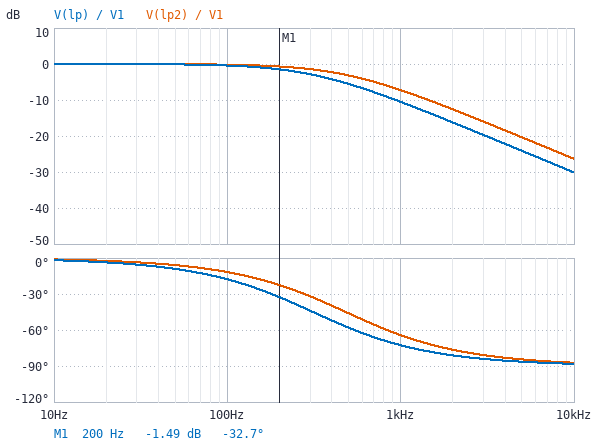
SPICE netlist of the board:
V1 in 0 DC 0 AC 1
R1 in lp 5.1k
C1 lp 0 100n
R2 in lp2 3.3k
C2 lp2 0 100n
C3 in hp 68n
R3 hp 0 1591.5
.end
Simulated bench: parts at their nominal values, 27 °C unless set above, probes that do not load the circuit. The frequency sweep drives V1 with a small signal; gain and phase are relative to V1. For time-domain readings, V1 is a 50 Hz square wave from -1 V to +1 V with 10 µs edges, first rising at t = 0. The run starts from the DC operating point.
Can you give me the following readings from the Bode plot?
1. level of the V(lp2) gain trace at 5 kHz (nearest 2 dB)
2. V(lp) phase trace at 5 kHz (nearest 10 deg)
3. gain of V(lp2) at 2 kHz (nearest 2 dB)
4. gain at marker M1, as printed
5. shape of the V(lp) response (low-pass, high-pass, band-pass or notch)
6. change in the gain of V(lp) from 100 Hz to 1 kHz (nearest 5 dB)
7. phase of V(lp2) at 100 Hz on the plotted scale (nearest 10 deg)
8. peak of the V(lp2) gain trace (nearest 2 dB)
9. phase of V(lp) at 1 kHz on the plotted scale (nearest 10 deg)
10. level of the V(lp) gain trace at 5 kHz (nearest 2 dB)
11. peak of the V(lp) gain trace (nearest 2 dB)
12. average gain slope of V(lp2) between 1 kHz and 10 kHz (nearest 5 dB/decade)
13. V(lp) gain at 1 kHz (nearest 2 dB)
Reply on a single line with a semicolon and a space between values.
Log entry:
-20 dB; -90 deg; -12 dB; -1.49 dB; low-pass; -10 dB; -10 deg; 0 dB; -70 deg; -24 dB; 0 dB; -20 dB/decade; -10 dB
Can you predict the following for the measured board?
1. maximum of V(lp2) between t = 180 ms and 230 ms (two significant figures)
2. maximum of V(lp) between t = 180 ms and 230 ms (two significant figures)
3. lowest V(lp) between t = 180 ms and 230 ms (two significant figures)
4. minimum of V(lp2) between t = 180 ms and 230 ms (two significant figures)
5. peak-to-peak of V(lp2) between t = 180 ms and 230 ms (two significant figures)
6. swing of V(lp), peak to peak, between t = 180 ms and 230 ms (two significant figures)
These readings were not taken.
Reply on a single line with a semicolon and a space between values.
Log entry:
1.0 V; 1.0 V; -1.0 V; -1.0 V; 2.0 V; 2.0 V
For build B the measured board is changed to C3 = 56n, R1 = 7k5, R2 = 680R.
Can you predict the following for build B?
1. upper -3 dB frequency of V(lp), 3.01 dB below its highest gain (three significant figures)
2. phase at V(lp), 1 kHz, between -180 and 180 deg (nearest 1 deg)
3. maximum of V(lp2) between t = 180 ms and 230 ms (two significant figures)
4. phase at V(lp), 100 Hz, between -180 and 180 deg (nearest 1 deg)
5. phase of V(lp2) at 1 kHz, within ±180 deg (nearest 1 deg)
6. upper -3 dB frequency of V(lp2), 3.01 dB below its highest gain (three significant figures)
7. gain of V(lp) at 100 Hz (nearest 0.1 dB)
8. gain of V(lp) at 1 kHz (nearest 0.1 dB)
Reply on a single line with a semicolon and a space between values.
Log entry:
212 Hz; -78 deg; 1.0 V; -25 deg; -23 deg; 2.34 kHz; -0.9 dB; -13.7 dB
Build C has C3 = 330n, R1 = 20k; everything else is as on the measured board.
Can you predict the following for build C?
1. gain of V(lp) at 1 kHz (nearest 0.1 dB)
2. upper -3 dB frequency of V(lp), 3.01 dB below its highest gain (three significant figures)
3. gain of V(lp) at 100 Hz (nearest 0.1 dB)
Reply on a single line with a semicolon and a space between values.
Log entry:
-22.0 dB; 79.6 Hz; -4.1 dB
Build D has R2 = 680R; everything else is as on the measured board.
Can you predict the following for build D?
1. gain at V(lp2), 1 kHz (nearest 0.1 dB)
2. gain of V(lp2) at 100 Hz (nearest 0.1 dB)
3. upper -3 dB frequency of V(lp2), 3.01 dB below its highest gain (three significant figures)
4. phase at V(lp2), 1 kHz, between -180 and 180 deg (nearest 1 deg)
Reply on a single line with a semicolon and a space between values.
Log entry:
-0.7 dB; 0 dB; 2.34 kHz; -23 deg
